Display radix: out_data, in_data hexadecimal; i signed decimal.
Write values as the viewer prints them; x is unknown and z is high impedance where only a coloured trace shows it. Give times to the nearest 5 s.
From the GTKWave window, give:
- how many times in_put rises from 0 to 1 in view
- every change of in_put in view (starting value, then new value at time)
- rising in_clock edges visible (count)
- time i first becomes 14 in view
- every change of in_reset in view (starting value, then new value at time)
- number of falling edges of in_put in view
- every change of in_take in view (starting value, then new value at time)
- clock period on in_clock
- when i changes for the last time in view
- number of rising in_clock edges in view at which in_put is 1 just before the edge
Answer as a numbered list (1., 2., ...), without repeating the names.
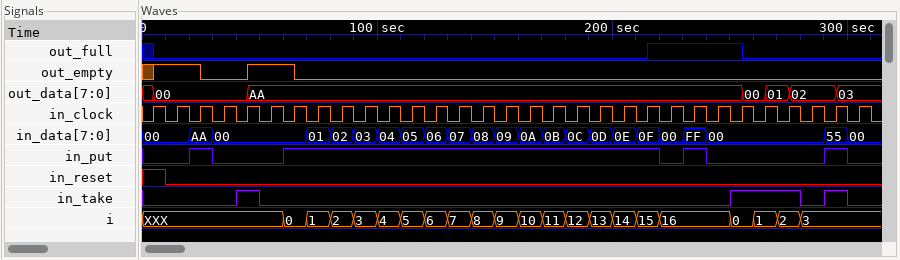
1. 4
2. 0, 1 at 20 s, 0 at 30 s, 1 at 60 s, 0 at 220 s, 1 at 230 s, 0 at 240 s, 1 at 290 s, 0 at 300 s
3. 31
4. 200 s
5. 1, 0 at 10 s
6. 4
7. 0, 1 at 40 s, 0 at 50 s, 1 at 250 s, 0 at 280 s, 1 at 290 s, 0 at 300 s
8. 10 s
9. 280 s
10. 19
